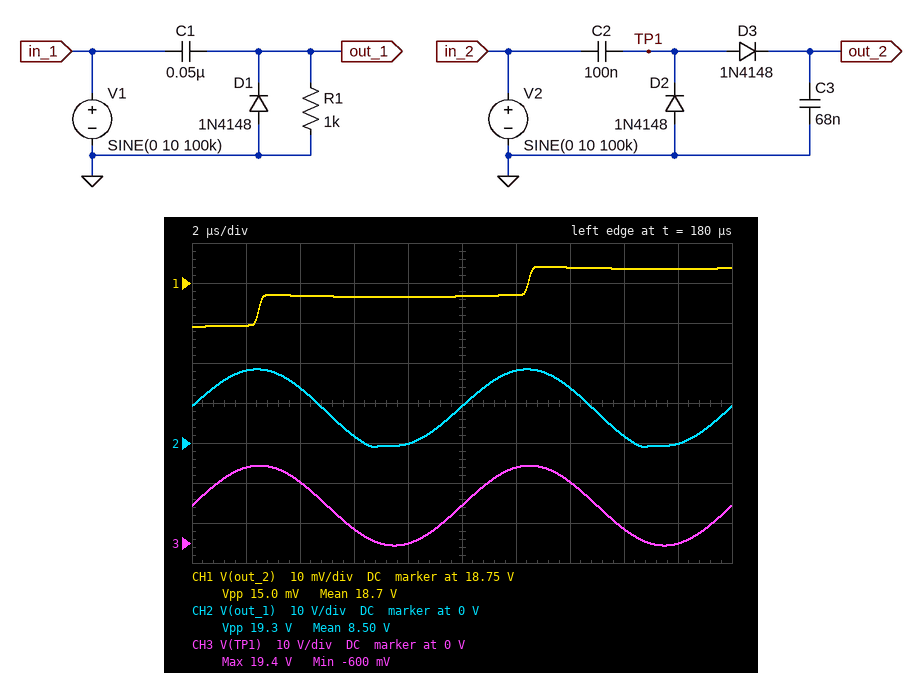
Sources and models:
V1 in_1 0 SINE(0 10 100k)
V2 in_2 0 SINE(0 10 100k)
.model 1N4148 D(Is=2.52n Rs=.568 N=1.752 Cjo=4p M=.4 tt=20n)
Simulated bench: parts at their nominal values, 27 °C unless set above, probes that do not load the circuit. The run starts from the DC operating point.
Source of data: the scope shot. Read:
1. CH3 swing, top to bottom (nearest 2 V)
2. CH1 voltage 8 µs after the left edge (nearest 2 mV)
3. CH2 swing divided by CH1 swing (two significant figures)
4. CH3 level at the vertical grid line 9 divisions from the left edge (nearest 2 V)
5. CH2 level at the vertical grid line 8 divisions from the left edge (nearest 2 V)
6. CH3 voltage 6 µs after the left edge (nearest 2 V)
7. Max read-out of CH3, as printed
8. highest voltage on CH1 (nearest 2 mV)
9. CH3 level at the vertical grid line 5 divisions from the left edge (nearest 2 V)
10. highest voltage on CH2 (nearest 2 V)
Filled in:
20 V
18.746 V
1300
0 V
2 V
4 V
19.4 V
18.754 V
10 V
18 V
